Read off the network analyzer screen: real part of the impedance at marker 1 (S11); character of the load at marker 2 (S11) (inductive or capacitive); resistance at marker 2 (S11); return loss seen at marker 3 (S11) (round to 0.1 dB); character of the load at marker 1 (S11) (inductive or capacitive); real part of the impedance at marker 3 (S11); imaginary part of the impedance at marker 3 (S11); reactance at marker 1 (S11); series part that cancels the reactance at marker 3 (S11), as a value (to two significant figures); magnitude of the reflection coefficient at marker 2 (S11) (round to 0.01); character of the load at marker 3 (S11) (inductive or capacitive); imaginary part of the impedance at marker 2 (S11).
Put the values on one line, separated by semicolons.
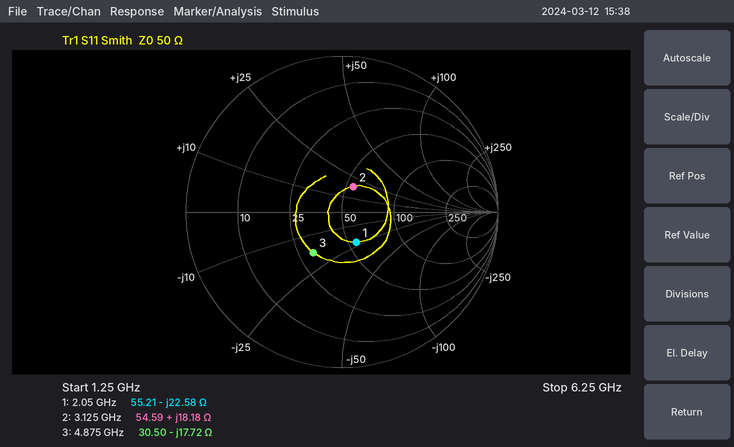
55.21 Ω; inductive; 54.59 Ω; 9.9 dB; capacitive; 30.50 Ω; -17.72 Ω; -22.58 Ω; 580 pH; 0.18; capacitive; +18.18 Ω
